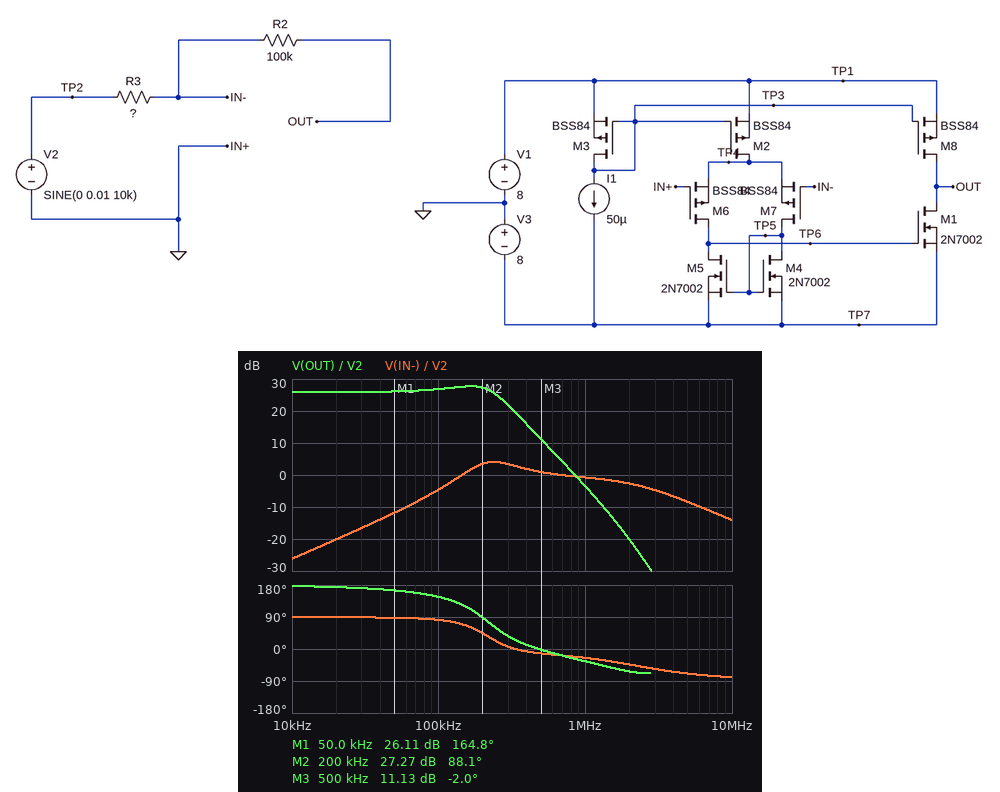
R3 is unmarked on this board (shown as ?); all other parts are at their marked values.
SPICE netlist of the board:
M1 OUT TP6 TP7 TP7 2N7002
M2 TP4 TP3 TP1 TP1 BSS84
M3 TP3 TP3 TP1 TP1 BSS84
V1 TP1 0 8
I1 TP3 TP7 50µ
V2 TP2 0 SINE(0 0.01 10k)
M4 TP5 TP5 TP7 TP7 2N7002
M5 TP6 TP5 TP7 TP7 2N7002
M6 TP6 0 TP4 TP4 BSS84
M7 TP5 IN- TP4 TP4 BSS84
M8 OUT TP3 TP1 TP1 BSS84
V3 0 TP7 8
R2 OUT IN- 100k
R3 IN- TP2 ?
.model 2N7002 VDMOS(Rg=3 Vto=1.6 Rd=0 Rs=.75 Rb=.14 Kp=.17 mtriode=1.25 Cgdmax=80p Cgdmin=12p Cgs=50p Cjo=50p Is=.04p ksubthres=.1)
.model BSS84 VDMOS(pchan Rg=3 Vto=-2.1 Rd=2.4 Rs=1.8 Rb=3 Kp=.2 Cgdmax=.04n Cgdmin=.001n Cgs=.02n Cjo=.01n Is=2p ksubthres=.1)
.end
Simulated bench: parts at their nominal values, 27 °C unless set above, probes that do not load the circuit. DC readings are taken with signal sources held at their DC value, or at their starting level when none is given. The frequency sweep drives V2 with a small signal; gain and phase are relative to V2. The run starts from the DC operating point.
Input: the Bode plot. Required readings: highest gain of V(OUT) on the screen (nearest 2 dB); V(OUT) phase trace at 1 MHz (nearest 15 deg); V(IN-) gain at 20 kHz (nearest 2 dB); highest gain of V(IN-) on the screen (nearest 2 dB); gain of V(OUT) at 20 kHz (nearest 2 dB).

28 dB
-30 deg
-20 dB
4 dB
26 dB
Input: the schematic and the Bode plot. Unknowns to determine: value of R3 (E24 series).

5.1 kΩ
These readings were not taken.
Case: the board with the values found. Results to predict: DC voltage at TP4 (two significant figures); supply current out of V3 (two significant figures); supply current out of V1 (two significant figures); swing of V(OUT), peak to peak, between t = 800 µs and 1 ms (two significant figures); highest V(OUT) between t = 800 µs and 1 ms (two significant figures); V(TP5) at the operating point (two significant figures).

1.9 V
150 µA
150 µA
390 mV
200 mV
-6.6 V
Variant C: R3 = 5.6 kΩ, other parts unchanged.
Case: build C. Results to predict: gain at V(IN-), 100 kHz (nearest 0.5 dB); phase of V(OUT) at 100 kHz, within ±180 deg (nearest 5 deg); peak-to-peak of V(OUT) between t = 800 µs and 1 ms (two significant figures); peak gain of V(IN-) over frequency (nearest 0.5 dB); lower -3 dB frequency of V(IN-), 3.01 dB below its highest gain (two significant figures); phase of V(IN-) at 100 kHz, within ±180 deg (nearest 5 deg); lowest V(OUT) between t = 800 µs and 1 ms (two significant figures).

-5.5 dB
150 deg
360 mV
4.5 dB
170 kHz
85 deg
-180 mV
